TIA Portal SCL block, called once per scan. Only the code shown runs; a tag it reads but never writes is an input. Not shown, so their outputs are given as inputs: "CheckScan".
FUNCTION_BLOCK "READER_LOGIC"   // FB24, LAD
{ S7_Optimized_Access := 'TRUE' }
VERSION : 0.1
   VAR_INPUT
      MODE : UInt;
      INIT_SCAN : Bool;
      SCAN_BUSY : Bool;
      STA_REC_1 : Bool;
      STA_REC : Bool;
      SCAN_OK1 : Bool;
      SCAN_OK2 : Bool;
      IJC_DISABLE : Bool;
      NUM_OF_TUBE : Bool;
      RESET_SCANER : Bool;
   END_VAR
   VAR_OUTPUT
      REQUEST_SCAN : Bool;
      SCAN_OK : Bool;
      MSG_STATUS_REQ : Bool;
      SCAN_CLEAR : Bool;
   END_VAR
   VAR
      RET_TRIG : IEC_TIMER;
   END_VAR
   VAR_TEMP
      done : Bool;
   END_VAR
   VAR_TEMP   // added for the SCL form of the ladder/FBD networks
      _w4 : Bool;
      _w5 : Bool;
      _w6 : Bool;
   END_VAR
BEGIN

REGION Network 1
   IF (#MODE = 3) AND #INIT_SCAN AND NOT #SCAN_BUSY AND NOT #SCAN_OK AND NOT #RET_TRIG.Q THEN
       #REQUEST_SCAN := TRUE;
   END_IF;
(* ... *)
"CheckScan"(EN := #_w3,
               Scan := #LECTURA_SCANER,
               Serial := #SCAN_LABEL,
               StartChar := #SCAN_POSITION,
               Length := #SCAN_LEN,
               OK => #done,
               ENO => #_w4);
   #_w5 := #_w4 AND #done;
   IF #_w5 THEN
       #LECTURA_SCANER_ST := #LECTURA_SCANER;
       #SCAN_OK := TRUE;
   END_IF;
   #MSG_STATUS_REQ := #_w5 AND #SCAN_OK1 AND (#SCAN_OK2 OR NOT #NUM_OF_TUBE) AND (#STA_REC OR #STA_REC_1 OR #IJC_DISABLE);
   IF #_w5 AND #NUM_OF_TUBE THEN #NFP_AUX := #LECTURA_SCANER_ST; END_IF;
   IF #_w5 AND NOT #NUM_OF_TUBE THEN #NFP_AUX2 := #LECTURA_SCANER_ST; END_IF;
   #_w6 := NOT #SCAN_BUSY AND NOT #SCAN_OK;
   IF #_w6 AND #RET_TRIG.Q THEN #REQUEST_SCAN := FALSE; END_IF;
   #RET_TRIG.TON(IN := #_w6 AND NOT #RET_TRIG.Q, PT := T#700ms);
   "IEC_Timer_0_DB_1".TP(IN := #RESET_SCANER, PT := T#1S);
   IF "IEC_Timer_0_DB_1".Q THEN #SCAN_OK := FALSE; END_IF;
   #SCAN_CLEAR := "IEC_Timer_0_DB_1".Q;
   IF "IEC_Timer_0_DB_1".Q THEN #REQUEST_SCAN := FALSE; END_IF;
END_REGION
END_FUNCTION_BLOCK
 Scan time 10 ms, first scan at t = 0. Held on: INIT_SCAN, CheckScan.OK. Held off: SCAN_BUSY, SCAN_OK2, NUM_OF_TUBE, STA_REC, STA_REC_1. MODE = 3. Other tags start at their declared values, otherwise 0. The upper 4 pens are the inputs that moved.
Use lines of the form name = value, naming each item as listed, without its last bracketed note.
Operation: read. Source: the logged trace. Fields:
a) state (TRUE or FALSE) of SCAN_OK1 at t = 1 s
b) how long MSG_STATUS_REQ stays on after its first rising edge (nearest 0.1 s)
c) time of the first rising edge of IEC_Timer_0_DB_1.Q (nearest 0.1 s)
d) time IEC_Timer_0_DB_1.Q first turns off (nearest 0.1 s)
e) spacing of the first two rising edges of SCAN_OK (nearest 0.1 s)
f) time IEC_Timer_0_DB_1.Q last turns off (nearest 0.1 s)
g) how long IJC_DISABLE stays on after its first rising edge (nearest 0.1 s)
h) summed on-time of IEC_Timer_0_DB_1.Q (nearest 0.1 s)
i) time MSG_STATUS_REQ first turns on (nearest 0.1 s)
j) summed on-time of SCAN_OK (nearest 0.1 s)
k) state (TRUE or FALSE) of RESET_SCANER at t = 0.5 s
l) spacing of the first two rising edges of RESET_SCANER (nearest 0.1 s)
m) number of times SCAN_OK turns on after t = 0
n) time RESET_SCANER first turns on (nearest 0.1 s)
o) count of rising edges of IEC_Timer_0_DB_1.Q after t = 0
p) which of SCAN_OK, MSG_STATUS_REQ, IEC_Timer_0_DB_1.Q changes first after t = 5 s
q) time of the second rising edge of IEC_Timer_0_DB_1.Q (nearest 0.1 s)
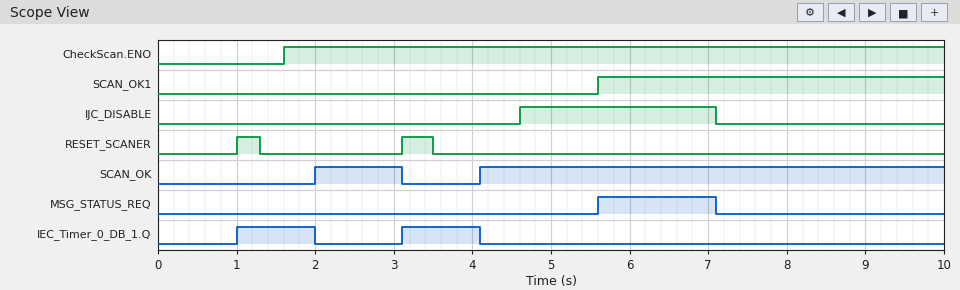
state (TRUE or FALSE) of SCAN_OK1 at t = 1 s = FALSE
how long MSG_STATUS_REQ stays on after its first rising edge = 1.5 s
time of the first rising edge of IEC_Timer_0_DB_1.Q = 1.0 s
time IEC_Timer_0_DB_1.Q first turns off = 2.0 s
spacing of the first two rising edges of SCAN_OK = 2.1 s
time IEC_Timer_0_DB_1.Q last turns off = 4.1 s
how long IJC_DISABLE stays on after its first rising edge = 2.5 s
summed on-time of IEC_Timer_0_DB_1.Q = 2.0 s
time MSG_STATUS_REQ first turns on = 5.6 s
summed on-time of SCAN_OK = 7.0 s
state (TRUE or FALSE) of RESET_SCANER at t = 0.5 s = FALSE
spacing of the first two rising edges of RESET_SCANER = 2.1 s
number of times SCAN_OK turns on after t = 0 = 2
time RESET_SCANER first turns on = 1.0 s
count of rising edges of IEC_Timer_0_DB_1.Q after t = 0 = 2
which of SCAN_OK, MSG_STATUS_REQ, IEC_Timer_0_DB_1.Q changes first after t = 5 s = MSG_STATUS_REQ
time of the second rising edge of IEC_Timer_0_DB_1.Q = 3.1 s
